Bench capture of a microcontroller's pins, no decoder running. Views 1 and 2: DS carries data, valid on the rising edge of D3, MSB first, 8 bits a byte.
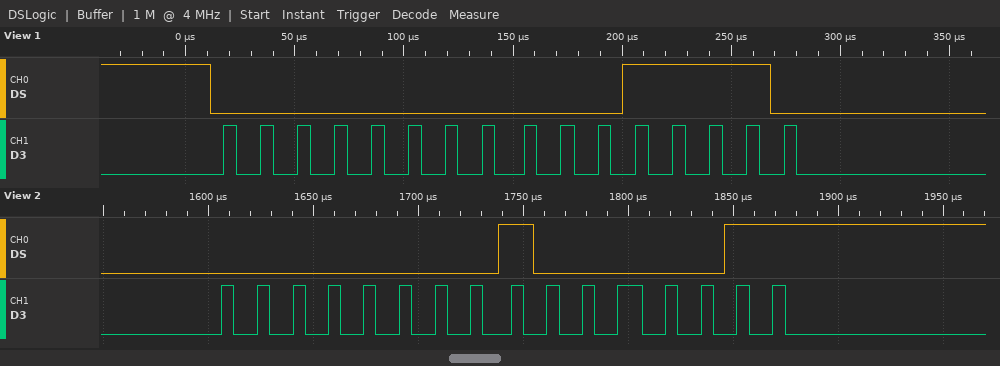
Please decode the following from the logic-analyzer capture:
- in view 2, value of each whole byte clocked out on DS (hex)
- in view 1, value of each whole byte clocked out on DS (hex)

00 83
00 1E
